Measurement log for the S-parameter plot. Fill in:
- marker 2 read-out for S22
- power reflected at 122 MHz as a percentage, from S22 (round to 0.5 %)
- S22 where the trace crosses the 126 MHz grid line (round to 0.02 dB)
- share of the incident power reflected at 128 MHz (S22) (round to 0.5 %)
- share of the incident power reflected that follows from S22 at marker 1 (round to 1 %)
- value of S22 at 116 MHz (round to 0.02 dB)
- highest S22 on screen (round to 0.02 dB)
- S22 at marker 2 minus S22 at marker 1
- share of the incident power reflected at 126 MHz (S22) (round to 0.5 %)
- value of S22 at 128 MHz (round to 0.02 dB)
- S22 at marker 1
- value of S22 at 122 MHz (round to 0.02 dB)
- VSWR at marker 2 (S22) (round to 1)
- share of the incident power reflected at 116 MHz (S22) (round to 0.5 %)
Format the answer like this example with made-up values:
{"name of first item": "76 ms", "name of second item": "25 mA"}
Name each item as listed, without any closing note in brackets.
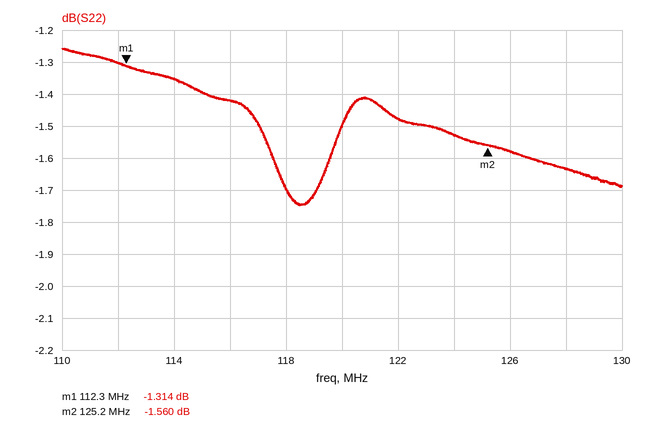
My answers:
{"marker 2 read-out for S22": "-1.560 dB", "power reflected at 122 MHz as a percentage, from S22": "71.0 %", "S22 where the trace crosses the 126 MHz grid line": "-1.58 dB", "share of the incident power reflected at 128 MHz (S22)": "68.5 %", "share of the incident power reflected that follows from S22 at marker 1": "74 %", "value of S22 at 116 MHz": "-1.42 dB", "highest S22 on screen": "-1.26 dB", "S22 at marker 2 minus S22 at marker 1": "-0.246 dB", "share of the incident power reflected at 126 MHz (S22)": "69.5 %", "value of S22 at 128 MHz": "-1.64 dB", "S22 at marker 1": "-1.314 dB", "value of S22 at 122 MHz": "-1.48 dB", "VSWR at marker 2 (S22)": "11", "share of the incident power reflected at 116 MHz (S22)": "72.0 %"}
